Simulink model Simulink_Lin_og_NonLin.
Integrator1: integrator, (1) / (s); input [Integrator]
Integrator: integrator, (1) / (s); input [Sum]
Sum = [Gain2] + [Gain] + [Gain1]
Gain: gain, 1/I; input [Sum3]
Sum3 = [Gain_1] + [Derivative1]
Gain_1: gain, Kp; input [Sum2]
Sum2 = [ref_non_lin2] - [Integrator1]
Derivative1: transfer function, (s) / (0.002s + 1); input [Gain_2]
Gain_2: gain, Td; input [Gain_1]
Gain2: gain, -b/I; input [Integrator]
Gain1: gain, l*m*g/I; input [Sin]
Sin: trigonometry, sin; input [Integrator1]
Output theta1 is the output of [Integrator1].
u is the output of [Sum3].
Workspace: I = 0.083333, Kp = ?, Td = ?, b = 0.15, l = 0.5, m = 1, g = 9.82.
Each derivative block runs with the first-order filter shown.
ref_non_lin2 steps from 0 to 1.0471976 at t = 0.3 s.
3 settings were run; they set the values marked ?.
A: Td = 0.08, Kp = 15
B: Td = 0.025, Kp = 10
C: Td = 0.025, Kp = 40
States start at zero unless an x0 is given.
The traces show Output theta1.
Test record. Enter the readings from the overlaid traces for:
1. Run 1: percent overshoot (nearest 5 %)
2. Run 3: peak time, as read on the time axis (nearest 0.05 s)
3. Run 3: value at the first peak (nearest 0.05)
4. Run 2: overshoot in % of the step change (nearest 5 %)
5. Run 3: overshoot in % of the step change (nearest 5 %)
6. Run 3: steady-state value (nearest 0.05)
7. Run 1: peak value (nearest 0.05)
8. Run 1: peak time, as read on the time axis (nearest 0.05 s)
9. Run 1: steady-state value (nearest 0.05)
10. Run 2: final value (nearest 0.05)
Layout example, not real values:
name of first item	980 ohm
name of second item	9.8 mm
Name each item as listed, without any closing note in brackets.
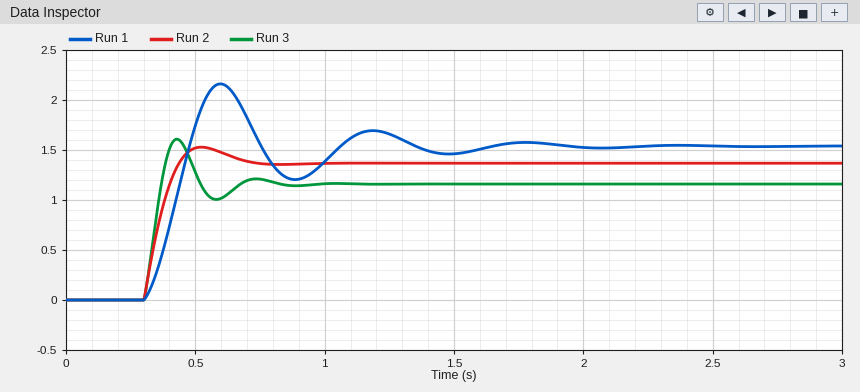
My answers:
Run 1: percent overshoot	40 %
Run 3: peak time, as read on the time axis	0.45 s
Run 3: value at the first peak	1.60
Run 2: overshoot in % of the step change	10 %
Run 3: overshoot in % of the step change	40 %
Run 3: steady-state value	1.15
Run 1: peak value	2.15
Run 1: peak time, as read on the time axis	0.60 s
Run 1: steady-state value	1.55
Run 2: final value	1.35
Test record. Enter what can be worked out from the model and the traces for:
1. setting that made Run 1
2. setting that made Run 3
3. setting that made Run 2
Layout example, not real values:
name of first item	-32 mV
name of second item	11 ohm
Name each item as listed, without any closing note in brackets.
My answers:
setting that made Run 1	B
setting that made Run 3	C
setting that made Run 2	A
